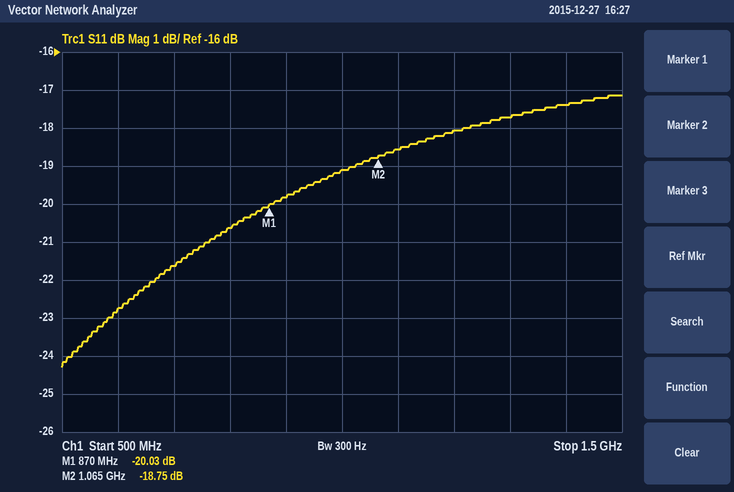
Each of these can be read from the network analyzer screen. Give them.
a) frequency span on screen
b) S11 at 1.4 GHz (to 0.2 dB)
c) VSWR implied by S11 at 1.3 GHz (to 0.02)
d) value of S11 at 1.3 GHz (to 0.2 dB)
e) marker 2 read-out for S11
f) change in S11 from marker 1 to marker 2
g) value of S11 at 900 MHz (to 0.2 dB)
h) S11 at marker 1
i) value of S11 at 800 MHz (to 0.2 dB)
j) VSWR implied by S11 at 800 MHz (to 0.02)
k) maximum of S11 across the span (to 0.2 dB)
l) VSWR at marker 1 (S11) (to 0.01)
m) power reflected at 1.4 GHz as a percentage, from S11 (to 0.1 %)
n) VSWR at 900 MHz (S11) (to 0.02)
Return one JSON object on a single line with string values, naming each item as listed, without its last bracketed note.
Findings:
{"frequency span on screen": "1 GHz", "S11 at 1.4 GHz": "-17.4 dB", "VSWR implied by S11 at 1.3 GHz": "1.30", "value of S11 at 1.3 GHz": "-17.8 dB", "marker 2 read-out for S11": "-18.75 dB", "change in S11 from marker 1 to marker 2": "1.28 dB", "value of S11 at 900 MHz": "-19.8 dB", "S11 at marker 1": "-20.03 dB", "value of S11 at 800 MHz": "-20.6 dB", "VSWR implied by S11 at 800 MHz": "1.20", "maximum of S11 across the span": "-17.2 dB", "VSWR at marker 1 (S11)": "1.22", "power reflected at 1.4 GHz as a percentage, from S11": "1.8 %", "VSWR at 900 MHz (S11)": "1.22"}
